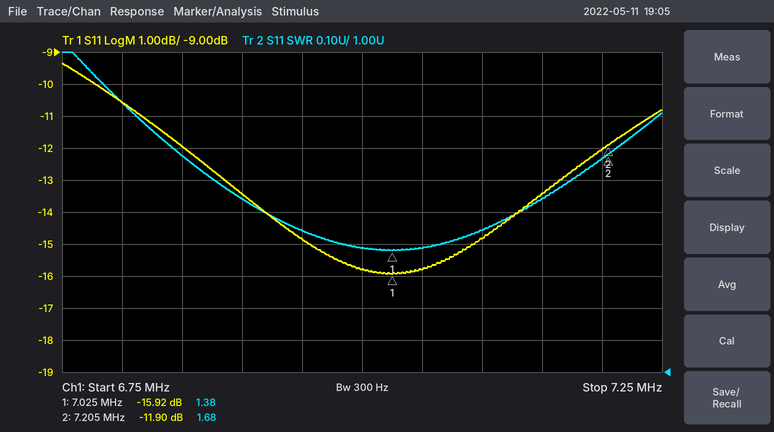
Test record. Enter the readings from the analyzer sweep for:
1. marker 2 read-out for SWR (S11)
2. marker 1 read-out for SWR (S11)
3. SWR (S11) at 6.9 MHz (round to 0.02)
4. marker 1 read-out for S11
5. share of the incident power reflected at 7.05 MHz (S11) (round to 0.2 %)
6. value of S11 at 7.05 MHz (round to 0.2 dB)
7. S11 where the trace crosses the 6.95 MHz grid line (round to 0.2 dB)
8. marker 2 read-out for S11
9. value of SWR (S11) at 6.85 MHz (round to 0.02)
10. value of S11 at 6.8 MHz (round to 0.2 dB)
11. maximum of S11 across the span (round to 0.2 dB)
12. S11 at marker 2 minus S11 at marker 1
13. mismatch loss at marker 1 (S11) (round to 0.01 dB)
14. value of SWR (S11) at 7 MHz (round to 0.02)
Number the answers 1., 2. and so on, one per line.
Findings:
1. 1.68
2. 1.38
3. 1.54
4. -15.92 dB
5. 2.6 %
6. -15.8 dB
7. -14.8 dB
8. -11.90 dB
9. 1.68
10. -10.6 dB
11. -9.4 dB
12. 4.02 dB
13. 0.11 dB
14. 1.38
